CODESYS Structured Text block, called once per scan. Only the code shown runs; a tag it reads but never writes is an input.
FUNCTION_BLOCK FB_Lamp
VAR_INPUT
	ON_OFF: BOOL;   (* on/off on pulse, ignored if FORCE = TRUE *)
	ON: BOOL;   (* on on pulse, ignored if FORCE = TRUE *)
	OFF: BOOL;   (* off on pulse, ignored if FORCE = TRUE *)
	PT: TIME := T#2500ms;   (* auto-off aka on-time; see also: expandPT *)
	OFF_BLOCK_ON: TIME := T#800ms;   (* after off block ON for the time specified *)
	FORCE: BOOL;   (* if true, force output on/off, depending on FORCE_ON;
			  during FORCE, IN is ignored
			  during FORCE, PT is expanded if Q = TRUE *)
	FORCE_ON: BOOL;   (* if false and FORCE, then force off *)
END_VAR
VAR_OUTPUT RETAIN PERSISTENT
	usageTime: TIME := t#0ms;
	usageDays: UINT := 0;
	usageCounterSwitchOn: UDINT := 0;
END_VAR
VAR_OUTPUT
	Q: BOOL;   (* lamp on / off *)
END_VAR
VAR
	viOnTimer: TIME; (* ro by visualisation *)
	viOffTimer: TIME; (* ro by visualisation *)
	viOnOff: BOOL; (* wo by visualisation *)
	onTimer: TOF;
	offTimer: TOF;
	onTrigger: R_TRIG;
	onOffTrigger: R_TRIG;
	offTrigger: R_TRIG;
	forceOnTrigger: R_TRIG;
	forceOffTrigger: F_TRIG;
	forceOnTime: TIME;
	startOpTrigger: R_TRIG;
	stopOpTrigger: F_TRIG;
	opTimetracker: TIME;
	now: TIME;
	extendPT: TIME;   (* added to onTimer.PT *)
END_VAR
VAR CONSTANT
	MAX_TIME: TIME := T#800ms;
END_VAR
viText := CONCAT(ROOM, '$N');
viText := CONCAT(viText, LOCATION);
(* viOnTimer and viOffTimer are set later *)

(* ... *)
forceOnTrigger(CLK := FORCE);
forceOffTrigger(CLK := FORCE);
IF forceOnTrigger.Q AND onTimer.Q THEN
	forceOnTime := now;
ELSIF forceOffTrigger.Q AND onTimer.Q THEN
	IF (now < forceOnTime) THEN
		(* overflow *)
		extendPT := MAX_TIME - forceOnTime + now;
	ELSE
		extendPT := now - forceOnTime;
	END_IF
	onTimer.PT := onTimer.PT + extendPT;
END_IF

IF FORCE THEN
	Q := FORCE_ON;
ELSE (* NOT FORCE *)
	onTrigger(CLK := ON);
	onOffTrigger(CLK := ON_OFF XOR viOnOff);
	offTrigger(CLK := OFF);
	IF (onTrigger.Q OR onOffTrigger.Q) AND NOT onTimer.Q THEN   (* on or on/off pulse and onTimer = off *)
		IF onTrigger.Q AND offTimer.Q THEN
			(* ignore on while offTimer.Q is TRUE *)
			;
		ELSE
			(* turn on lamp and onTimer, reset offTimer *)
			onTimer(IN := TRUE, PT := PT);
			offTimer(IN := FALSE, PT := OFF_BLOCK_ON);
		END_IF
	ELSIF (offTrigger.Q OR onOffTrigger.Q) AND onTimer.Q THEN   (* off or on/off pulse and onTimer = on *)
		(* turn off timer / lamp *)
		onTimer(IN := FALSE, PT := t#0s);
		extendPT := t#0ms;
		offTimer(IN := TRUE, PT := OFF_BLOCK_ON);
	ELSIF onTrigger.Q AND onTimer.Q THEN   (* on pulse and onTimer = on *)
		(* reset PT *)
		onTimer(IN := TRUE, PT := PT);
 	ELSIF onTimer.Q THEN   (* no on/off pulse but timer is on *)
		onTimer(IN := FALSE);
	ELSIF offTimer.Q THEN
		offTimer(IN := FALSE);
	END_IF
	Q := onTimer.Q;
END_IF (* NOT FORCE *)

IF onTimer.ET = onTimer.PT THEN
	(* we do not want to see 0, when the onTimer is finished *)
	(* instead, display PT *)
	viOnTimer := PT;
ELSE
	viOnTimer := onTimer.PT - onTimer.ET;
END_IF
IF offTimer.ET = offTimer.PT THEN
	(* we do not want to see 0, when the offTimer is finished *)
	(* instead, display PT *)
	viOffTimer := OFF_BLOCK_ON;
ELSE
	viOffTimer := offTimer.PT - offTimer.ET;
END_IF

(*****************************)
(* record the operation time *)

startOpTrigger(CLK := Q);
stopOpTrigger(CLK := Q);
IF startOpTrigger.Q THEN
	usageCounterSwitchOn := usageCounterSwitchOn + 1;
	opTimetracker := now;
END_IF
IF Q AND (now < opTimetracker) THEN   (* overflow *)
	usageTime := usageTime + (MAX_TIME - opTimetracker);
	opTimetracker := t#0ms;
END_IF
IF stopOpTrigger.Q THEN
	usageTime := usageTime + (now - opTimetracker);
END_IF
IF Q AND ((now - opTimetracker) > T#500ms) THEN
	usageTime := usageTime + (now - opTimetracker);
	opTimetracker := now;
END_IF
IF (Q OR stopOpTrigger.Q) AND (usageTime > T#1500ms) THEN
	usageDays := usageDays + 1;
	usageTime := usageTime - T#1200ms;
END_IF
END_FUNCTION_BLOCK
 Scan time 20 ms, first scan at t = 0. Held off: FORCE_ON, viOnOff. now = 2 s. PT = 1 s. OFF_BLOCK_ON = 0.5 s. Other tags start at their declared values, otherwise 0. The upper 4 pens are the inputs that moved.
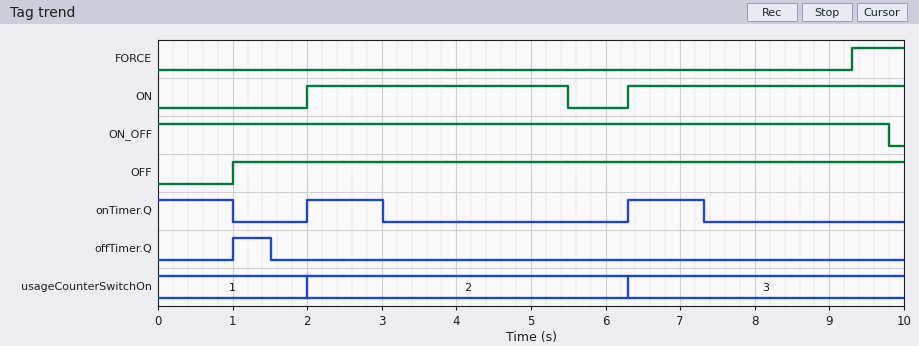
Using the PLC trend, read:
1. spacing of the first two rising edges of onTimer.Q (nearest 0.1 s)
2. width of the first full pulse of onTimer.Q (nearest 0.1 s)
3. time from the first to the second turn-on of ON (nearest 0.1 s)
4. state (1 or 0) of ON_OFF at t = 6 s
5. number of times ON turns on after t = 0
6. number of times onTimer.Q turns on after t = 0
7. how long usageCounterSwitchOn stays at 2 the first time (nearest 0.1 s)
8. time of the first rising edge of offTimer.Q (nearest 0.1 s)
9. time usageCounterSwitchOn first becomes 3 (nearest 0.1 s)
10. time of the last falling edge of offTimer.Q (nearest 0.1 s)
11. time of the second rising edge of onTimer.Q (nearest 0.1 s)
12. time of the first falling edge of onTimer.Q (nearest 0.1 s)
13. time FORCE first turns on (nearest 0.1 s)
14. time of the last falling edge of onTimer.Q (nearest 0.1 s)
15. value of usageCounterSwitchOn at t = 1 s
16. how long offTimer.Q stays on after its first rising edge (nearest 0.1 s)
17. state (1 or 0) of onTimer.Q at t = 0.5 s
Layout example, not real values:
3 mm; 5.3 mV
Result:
4.3 s; 1.0 s; 4.3 s; 1; 2; 2; 4.3 s; 1.0 s; 6.3 s; 1.5 s; 6.3 s; 1.0 s; 9.3 s; 7.3 s; 1; 0.5 s; 1
